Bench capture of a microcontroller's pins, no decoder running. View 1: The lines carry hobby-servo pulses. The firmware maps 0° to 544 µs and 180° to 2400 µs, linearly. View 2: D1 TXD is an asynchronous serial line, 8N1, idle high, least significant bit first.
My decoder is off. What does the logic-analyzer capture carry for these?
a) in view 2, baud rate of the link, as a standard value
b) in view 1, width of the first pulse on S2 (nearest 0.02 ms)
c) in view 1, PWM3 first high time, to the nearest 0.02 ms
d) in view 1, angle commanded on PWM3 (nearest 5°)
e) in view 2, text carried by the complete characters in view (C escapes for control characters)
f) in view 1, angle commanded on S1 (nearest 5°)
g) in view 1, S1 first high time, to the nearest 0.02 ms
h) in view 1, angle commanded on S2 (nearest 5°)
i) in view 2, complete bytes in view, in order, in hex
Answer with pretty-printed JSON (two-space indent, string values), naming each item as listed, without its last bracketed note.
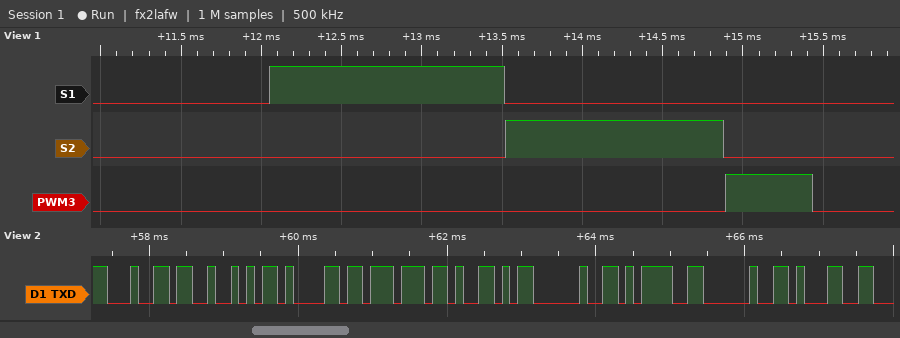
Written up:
{
  "in view 2, baud rate of the link, as a standard value": "9600 baud",
  "in view 1, width of the first pulse on S2": "1.36 ms",
  "in view 1, PWM3 first high time, to the nearest 0.02 ms": "0.54 ms",
  "in view 1, angle commanded on PWM3": "0°",
  "in view 2, text carried by the complete characters in view": "\"dRawY = 1\"",
  "in view 1, angle commanded on S1": "90°",
  "in view 1, S1 first high time, to the nearest 0.02 ms": "1.46 ms",
  "in view 1, angle commanded on S2": "80°",
  "in view 2, complete bytes in view, in order, in hex": "64 52 61 77 59 20 3D 20 31"
}
